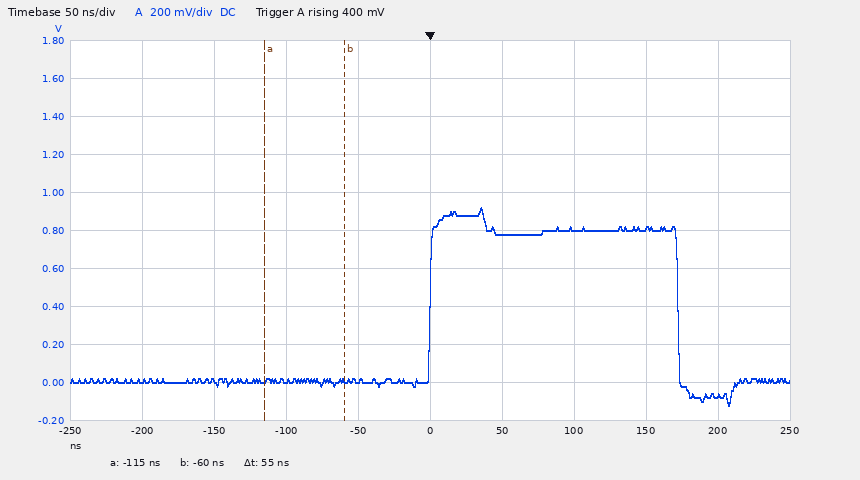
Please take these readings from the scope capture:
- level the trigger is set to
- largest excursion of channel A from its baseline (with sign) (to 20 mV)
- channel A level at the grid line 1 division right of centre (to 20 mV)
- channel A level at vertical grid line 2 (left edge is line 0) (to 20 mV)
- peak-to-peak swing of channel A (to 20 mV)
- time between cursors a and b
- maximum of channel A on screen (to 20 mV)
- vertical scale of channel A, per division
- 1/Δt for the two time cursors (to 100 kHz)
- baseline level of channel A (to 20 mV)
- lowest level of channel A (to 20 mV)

400 mV
+920 mV
780 mV
0 mV
1.04 V
55 ns
920 mV
200 mV
18.2 MHz
0 mV
-120 mV
